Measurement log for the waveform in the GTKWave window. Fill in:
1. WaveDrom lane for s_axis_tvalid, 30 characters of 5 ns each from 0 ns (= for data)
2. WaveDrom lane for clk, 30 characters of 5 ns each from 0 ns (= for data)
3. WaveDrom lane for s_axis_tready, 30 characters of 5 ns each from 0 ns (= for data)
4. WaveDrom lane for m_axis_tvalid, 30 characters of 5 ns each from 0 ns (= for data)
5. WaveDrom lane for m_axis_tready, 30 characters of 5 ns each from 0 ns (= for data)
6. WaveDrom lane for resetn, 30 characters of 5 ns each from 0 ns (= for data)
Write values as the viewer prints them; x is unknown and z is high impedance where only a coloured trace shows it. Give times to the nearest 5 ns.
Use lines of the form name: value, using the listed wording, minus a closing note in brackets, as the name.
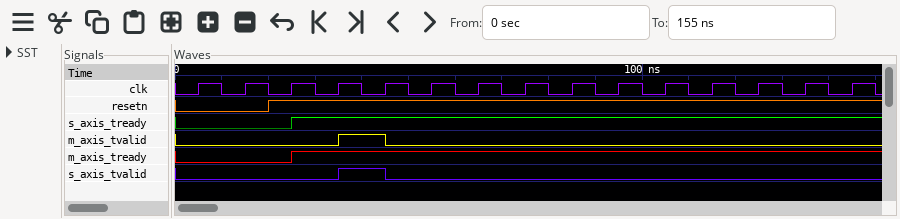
WaveDrom lane for s_axis_tvalid, 30 characters of 5 ns each from 0 ns: {name: 's_axis_tvalid', wave: '0......1.0....................'}
WaveDrom lane for clk, 30 characters of 5 ns each from 0 ns: {name: 'clk', wave: '010101010101010101010101010101'}
WaveDrom lane for s_axis_tready, 30 characters of 5 ns each from 0 ns: {name: 's_axis_tready', wave: '0....1........................'}
WaveDrom lane for m_axis_tvalid, 30 characters of 5 ns each from 0 ns: {name: 'm_axis_tvalid', wave: '0......1.0....................'}
WaveDrom lane for m_axis_tready, 30 characters of 5 ns each from 0 ns: {name: 'm_axis_tready', wave: '0....1........................'}
WaveDrom lane for resetn, 30 characters of 5 ns each from 0 ns: {name: 'resetn', wave: '0...1.........................'}
